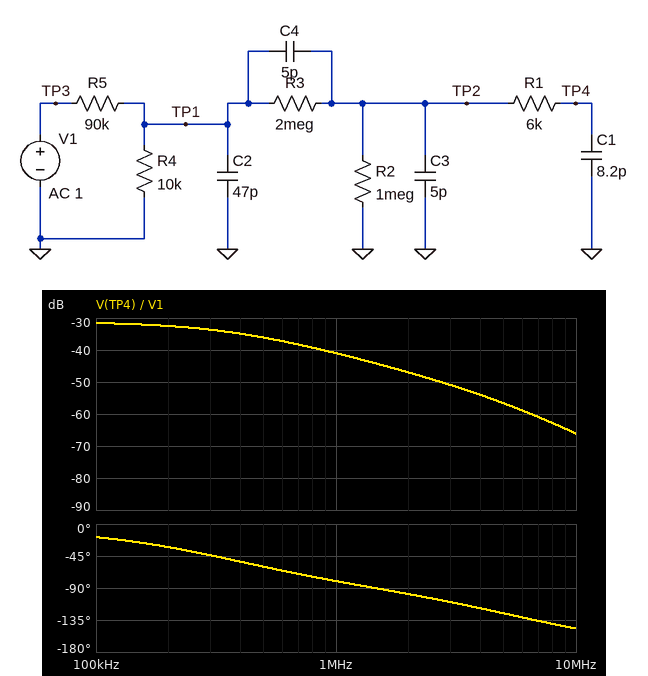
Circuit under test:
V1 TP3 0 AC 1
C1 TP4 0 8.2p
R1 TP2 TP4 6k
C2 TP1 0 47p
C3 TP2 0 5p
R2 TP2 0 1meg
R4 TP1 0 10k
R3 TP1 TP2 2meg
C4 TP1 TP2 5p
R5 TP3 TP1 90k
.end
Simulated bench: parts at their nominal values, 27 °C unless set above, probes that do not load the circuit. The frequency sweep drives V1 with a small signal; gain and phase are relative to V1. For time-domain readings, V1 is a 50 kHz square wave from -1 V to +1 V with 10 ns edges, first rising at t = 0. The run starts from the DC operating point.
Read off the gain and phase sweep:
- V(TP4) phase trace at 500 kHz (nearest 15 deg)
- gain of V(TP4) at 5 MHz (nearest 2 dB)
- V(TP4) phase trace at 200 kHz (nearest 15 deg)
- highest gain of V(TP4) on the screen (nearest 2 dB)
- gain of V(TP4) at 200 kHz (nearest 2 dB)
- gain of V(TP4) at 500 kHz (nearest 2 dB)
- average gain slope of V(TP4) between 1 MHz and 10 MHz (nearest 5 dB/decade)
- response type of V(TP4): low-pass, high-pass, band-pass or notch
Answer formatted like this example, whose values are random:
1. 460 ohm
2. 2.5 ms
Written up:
1. -60 deg
2. -56 dB
3. -30 deg
4. -32 dB
5. -32 dB
6. -36 dB
7. -25 dB/decade
8. low-pass
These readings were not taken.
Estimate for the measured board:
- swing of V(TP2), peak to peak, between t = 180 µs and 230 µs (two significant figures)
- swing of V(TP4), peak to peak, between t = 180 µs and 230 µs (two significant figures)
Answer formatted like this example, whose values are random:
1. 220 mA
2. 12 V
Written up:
1. 59 mV
2. 59 mV
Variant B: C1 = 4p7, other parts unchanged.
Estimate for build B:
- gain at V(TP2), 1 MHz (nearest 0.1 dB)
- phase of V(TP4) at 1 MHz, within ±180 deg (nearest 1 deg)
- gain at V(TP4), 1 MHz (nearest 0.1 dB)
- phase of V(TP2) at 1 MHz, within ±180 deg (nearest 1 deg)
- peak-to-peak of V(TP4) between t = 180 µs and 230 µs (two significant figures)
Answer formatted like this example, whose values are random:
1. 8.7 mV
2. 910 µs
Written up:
1. -38.9 dB
2. -77 deg
3. -39.0 dB
4. -67 deg
5. 68 mV
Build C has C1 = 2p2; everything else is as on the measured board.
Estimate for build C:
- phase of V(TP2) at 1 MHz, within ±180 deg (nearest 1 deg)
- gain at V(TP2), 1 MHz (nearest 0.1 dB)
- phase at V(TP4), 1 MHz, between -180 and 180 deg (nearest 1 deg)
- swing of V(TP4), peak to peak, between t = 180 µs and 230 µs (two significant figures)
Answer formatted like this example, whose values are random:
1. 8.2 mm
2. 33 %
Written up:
1. -69 deg
2. -37.3 dB
3. -74 deg
4. 84 mV
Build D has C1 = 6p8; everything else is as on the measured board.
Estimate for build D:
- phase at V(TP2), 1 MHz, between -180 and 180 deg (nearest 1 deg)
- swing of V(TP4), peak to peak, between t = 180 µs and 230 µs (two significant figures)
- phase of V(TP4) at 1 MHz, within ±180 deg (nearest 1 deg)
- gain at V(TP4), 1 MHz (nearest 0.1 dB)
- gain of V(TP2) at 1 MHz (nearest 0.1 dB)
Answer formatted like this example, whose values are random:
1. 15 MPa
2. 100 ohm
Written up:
1. -65 deg
2. 62 mV
3. -79 deg
4. -40.3 dB
5. -40.0 dB
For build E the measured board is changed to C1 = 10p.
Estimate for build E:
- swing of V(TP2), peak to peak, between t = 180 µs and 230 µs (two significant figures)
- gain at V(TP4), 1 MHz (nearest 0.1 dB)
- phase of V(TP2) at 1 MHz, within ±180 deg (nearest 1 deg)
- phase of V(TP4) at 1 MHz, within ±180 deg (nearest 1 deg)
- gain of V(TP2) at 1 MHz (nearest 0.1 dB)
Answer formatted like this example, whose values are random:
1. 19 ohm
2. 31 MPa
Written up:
1. 55 mV
2. -41.9 dB
3. -61 deg
4. -81 deg
5. -41.3 dB
